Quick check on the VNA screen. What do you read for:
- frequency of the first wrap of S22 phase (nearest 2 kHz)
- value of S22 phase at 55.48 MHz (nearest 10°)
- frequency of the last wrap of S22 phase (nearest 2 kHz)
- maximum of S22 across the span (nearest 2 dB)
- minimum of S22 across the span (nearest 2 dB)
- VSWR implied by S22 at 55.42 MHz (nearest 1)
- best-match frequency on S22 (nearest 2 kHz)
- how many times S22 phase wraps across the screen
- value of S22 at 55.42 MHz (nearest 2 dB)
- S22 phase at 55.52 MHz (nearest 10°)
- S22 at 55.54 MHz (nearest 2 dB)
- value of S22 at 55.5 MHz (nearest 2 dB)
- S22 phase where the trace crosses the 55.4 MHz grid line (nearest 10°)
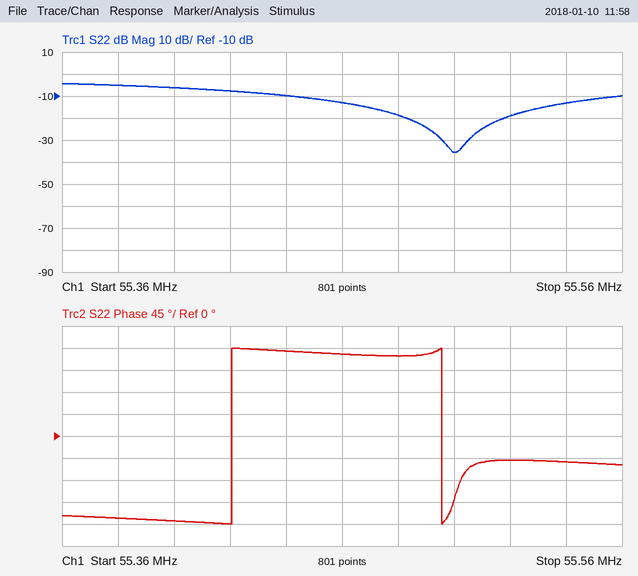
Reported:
55.420 MHz
160°
55.496 MHz
-4 dB
-36 dB
2
55.500 MHz
2
-8 dB
-50°
-14 dB
-36 dB
-170°
